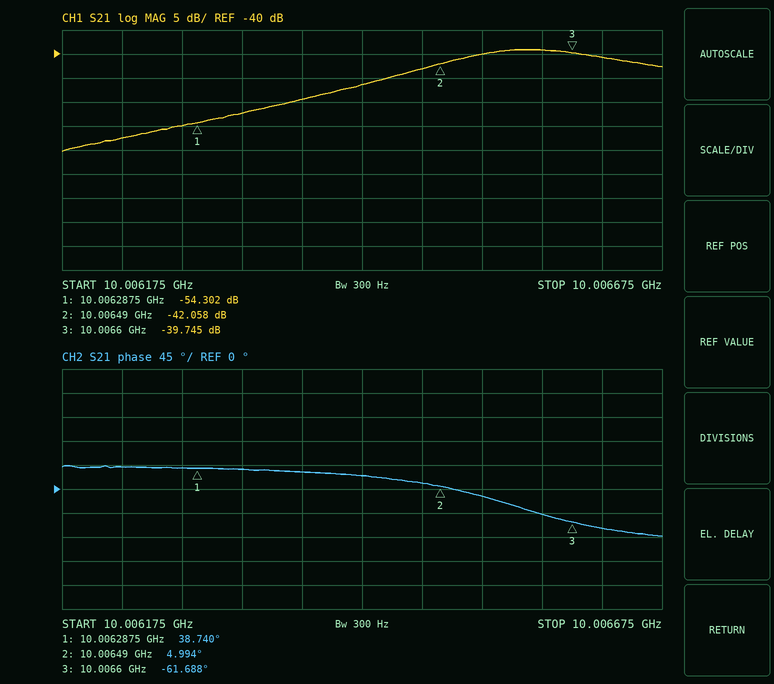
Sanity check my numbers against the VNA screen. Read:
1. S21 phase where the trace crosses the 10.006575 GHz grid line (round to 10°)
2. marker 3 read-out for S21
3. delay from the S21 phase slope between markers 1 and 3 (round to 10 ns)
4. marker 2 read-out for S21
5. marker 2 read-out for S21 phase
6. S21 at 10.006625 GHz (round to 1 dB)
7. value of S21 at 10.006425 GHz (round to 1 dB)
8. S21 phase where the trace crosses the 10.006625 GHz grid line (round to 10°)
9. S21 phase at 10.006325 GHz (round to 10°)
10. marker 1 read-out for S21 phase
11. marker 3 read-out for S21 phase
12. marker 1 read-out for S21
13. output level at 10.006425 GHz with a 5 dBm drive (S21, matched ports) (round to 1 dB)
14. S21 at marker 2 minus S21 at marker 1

-50°
-39.745 dB
890 ns
-42.058 dB
4.994°
-41 dB
-46 dB
-70°
40°
38.740°
-61.688°
-54.302 dB
-41 dBm
12.244 dB
